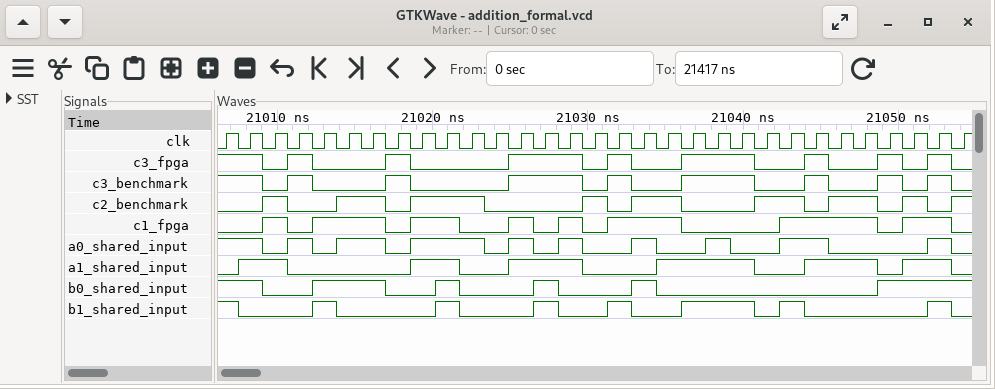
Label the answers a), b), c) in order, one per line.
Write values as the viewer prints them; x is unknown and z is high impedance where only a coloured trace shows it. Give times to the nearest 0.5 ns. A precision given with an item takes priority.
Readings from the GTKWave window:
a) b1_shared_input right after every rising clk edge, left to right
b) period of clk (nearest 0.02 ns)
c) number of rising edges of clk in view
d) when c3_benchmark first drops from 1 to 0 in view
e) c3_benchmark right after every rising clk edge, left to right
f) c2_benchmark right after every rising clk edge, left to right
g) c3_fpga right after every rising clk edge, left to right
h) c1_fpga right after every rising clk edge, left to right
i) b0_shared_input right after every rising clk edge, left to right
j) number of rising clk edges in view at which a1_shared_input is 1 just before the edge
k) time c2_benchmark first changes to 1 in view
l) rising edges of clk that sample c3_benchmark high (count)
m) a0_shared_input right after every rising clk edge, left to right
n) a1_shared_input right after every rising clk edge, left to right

a) 1 0 0 0 1 0 0 0 0 1 0 0 0 1 0 0 1 0 0 1 1 1 0 1 0 0 0 0 0 1 0
b) 1.58 ns
c) 31
d) 21009 ns
e) 1 1 0 1 0 0 0 1 0 0 0 0 1 1 1 0 1 0 0 1 1 1 0 0 1 0 0 1 0 1 0
f) 0 0 1 0 0 1 1 0 1 1 1 0 0 0 0 1 0 1 1 0 0 0 1 1 0 1 1 0 1 0 1
g) 1 1 0 1 0 0 0 1 0 0 0 0 1 1 1 0 1 0 0 1 1 1 0 0 1 0 0 1 0 1 0
h) 0 0 1 0 1 1 1 0 1 1 0 0 1 0 1 0 1 1 1 0 0 0 0 1 1 1 1 0 1 1 0
i) 1 1 0 0 1 1 1 0 0 1 0 0 0 1 0 0 0 1 0 0 0 0 0 0 0 0 0 1 1 1 1
j) 16
k) 21009 ns
l) 14
m) 1 1 0 1 0 1 1 0 1 1 1 0 1 0 1 0 0 1 0 0 1 0 0 1 1 0 0 0 0 1 0
n) 0 1 1 0 0 0 0 0 1 1 0 0 1 1 1 0 0 0 1 1 1 1 0 0 1 1 1 0 1 1 0
